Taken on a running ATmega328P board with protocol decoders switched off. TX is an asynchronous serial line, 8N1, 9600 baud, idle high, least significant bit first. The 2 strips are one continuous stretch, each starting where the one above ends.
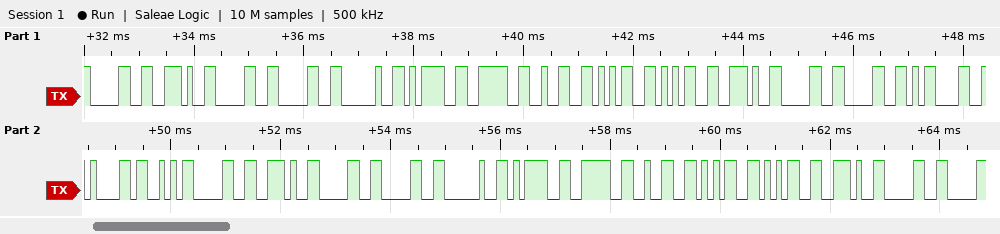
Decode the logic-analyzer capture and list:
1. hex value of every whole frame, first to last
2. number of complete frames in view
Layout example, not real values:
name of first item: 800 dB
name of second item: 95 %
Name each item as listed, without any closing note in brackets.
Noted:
hex value of every whole frame, first to last: 30 2E 30 30 20 3D 3E 32 35 35 2E 30 30 0D 0A 53 30 2E 30 30 20 3D 3E 32 35 35 2E 30
number of complete frames in view: 28
